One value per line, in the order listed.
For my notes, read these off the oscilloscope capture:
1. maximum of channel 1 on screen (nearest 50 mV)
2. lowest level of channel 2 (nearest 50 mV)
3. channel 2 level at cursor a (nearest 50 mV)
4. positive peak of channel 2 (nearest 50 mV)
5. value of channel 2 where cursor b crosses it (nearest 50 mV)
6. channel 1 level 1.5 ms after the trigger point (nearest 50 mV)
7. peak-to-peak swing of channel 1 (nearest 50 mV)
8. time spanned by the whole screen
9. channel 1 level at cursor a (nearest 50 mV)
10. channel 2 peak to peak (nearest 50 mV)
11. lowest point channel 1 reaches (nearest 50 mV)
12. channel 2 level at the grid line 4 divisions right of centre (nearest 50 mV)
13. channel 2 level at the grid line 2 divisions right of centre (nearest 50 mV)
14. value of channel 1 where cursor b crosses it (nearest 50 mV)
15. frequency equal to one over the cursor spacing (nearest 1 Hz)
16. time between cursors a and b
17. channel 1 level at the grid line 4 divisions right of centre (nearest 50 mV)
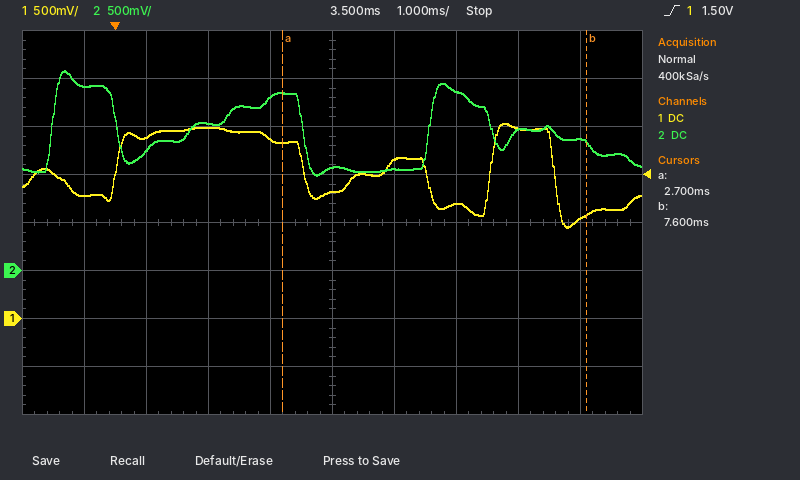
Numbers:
2.05 V
1.00 V
1.85 V
2.10 V
1.35 V
2.00 V
1.10 V
10 ms
1.85 V
1.10 V
950 mV
1.35 V
1.85 V
1.10 V
204 Hz
4.9 ms
1.05 V
